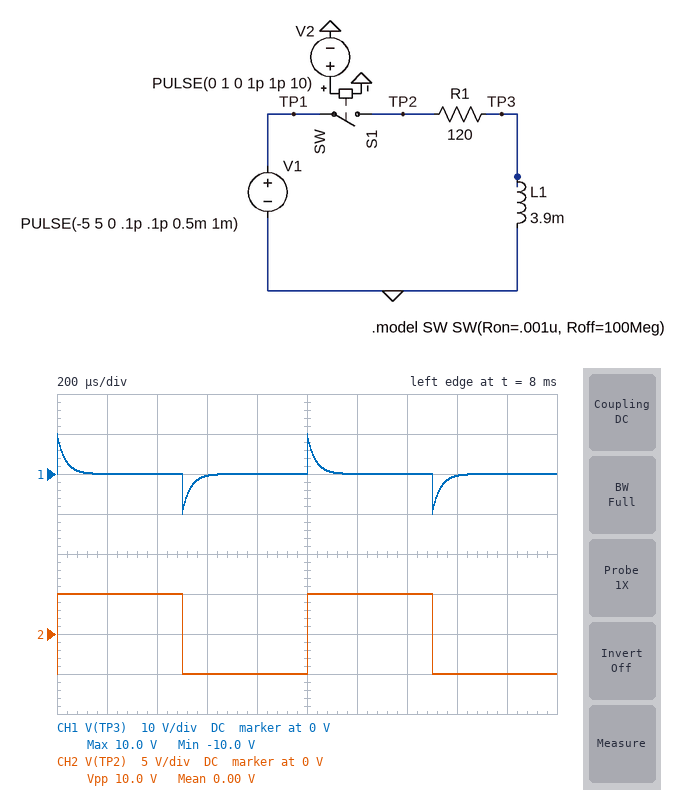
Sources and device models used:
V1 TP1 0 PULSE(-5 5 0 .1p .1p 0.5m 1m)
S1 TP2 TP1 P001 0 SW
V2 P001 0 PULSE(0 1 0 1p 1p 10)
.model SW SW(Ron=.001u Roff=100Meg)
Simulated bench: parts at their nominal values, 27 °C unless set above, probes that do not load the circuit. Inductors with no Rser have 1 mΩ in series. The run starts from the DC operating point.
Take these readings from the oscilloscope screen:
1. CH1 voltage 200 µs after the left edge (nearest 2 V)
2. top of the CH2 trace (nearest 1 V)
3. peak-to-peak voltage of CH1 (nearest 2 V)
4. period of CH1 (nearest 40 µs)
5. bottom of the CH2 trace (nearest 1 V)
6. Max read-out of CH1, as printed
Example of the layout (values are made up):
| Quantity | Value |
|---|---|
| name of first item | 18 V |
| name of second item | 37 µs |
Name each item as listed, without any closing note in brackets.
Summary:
| Quantity | Value |
|---|---|
| CH1 voltage 200 µs after the left edge | 0 V |
| top of the CH2 trace | 5 V |
| peak-to-peak voltage of CH1 | 20 V |
| period of CH1 | 1.00 ms |
| bottom of the CH2 trace | -5 V |
| Max read-out of CH1, as printed | 10.0 V |
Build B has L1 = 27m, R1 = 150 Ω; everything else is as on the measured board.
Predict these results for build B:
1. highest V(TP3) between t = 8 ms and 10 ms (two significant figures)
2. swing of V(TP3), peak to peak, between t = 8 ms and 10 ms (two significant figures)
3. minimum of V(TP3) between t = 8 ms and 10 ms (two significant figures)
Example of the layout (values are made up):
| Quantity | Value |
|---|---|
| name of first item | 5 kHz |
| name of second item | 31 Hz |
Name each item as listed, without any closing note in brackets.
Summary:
| Quantity | Value |
|---|---|
| highest V(TP3) between t = 8 ms and 10 ms | 9.4 V |
| swing of V(TP3), peak to peak, between t = 8 ms and 10 ms | 19 V |
| minimum of V(TP3) between t = 8 ms and 10 ms | -9.4 V |
